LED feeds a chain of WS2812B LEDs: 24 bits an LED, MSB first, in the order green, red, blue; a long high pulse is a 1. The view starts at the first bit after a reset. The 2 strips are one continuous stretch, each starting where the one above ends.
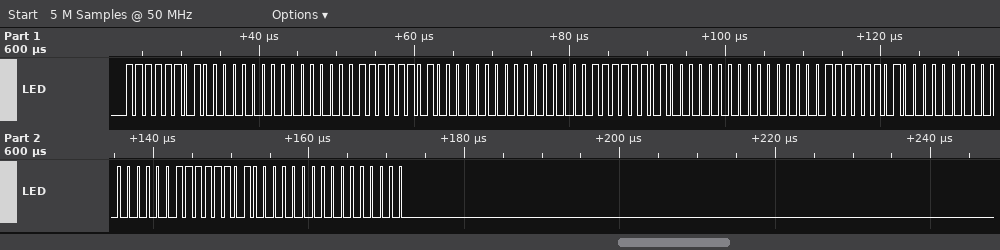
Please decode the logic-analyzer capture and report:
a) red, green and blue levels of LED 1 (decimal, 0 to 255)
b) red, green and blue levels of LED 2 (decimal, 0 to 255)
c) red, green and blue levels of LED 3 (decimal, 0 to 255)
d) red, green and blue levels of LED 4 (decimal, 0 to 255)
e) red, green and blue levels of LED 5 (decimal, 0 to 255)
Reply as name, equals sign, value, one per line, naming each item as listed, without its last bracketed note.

red, green and blue levels of LED 1 = 0, 253, 0
red, green and blue levels of LED 2 = 0, 253, 0
red, green and blue levels of LED 3 = 0, 253, 0
red, green and blue levels of LED 4 = 0, 253, 0
red, green and blue levels of LED 5 = 0, 253, 0
